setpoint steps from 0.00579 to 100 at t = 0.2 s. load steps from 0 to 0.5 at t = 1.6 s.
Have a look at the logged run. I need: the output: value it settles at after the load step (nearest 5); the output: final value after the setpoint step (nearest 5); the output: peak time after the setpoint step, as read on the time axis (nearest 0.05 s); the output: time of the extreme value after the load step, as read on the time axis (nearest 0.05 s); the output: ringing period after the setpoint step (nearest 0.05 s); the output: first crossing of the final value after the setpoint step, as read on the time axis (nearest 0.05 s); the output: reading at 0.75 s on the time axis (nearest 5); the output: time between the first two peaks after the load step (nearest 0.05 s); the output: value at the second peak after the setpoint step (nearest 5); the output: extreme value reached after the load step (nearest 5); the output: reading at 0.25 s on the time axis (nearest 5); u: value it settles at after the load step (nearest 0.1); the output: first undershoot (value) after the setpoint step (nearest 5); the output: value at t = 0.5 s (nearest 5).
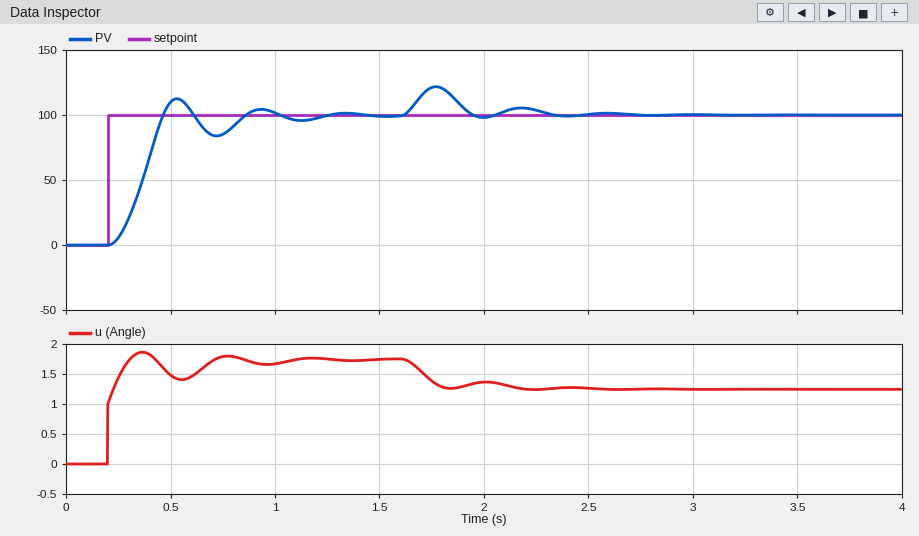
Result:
100
100
0.55 s
1.75 s
0.40 s
0.45 s
85
0.40 s
105
120
5
1.2
85
110
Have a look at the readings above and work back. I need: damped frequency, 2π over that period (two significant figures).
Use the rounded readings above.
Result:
16 rad/s
